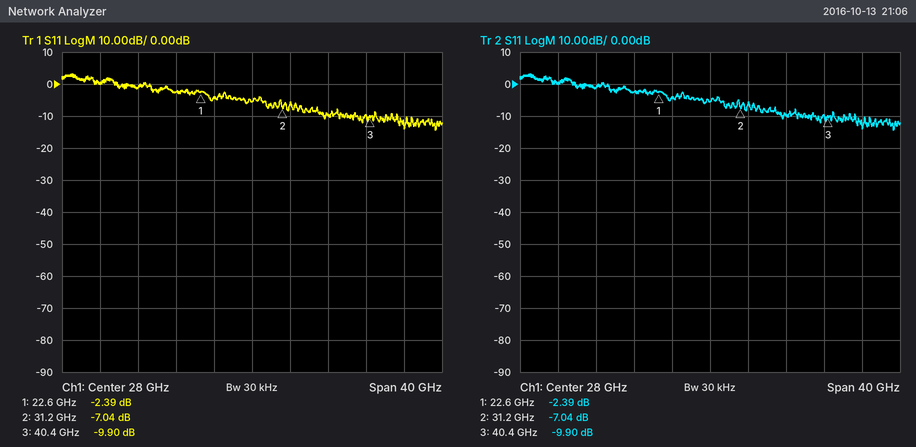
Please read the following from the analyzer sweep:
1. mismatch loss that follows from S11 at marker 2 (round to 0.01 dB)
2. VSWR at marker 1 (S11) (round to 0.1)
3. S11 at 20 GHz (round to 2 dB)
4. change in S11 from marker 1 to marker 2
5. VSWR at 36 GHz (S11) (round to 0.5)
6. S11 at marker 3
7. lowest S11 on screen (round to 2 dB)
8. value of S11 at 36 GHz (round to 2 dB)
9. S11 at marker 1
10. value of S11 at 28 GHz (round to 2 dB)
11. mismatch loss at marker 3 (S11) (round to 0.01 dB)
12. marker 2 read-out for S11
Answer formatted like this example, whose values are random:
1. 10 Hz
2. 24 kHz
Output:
1. 0.96 dB
2. 7.3
3. -2 dB
4. -4.65 dB
5. 2.0
6. -9.90 dB
7. -14 dB
8. -10 dB
9. -2.39 dB
10. -6 dB
11. 0.47 dB
12. -7.04 dB
